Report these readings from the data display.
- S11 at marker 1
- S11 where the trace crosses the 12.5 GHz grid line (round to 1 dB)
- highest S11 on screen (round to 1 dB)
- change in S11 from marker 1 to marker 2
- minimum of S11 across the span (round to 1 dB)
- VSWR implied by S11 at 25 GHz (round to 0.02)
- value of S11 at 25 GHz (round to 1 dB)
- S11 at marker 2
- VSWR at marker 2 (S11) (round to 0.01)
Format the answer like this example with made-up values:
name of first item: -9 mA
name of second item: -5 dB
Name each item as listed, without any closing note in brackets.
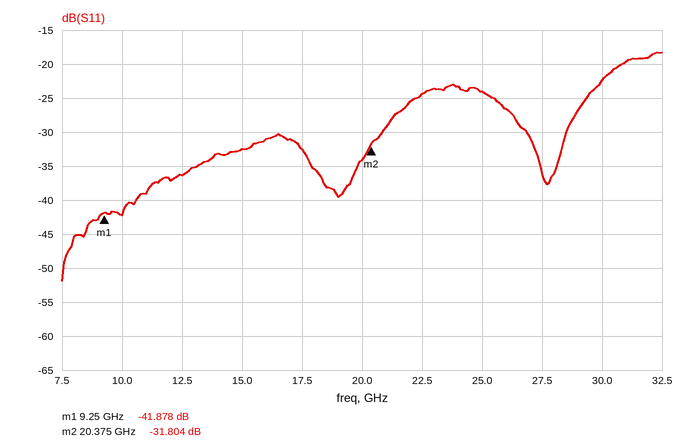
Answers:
S11 at marker 1: -41.878 dB
S11 where the trace crosses the 12.5 GHz grid line: -36 dB
highest S11 on screen: -18 dB
change in S11 from marker 1 to marker 2: 10.074 dB
minimum of S11 across the span: -52 dB
VSWR implied by S11 at 25 GHz: 1.14
value of S11 at 25 GHz: -24 dB
S11 at marker 2: -31.804 dB
VSWR at marker 2 (S11): 1.05
